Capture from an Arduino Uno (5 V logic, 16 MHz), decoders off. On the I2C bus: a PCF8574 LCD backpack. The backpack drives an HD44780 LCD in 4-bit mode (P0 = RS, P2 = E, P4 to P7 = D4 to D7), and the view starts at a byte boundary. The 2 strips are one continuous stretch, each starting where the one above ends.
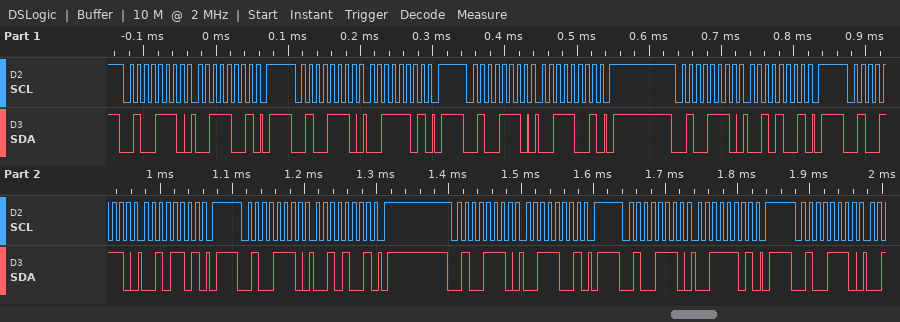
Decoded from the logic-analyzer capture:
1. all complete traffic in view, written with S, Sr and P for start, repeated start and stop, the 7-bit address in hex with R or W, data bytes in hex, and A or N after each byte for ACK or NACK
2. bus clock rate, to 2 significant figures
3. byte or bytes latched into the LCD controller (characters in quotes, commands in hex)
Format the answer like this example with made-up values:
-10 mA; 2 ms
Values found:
S 27W A 39 A P S 27W A 3D A P S 27W A 39 A P S 27W A 29 A P S 27W A 2D A P S 27W A 29 A P S 27W A 39 A P S 27W A 3D A P S 27W A; 100 kHz; '2'
